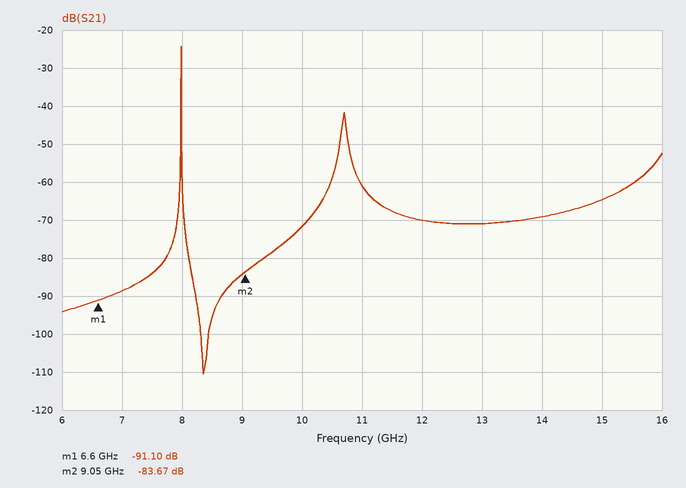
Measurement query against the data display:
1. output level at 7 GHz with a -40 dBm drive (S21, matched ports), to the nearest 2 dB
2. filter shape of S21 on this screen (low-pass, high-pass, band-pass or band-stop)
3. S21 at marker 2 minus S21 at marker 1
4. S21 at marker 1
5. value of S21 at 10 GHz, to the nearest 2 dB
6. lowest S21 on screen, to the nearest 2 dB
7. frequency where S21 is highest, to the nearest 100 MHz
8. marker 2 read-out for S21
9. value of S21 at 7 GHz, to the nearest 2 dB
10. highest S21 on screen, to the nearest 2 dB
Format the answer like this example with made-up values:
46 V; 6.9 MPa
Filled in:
-128 dBm; band-pass; 7.43 dB; -91.10 dB; -72 dB; -110 dB; 8.0 GHz; -83.67 dB; -88 dB; -24 dB
